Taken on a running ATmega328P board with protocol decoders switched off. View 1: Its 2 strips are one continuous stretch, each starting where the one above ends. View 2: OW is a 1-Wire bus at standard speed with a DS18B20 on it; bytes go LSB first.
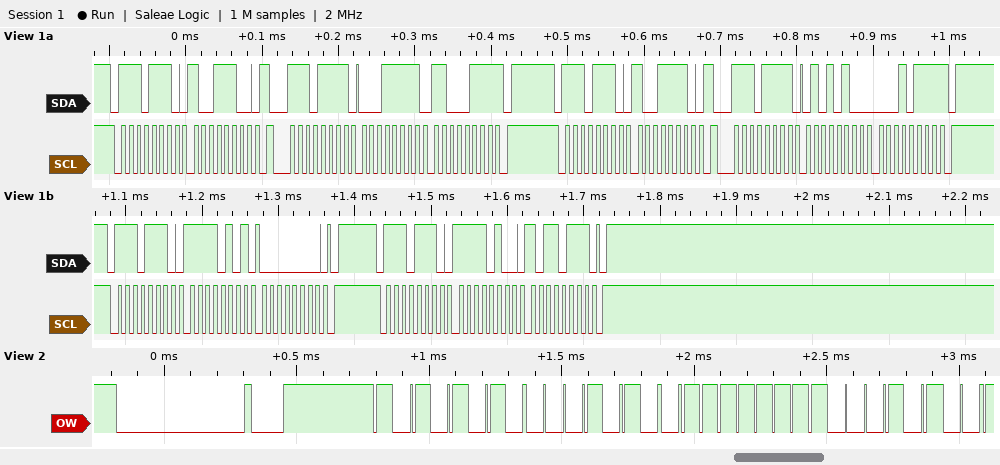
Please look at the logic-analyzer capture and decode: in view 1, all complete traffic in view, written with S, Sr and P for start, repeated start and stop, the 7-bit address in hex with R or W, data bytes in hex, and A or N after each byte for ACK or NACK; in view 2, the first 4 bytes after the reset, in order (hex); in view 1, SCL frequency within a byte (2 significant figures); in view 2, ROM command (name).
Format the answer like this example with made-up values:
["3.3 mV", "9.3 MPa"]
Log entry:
["S 77W A 9C A Sr 77R A 1F A C7 N P S 77W A 9E A Sr 77R A 54 A 17 N P S 77W A F5 A 00 A P S 77W A F4 A B7 A P", "55 28 FF 28", "100 kHz", "Match ROM"]
